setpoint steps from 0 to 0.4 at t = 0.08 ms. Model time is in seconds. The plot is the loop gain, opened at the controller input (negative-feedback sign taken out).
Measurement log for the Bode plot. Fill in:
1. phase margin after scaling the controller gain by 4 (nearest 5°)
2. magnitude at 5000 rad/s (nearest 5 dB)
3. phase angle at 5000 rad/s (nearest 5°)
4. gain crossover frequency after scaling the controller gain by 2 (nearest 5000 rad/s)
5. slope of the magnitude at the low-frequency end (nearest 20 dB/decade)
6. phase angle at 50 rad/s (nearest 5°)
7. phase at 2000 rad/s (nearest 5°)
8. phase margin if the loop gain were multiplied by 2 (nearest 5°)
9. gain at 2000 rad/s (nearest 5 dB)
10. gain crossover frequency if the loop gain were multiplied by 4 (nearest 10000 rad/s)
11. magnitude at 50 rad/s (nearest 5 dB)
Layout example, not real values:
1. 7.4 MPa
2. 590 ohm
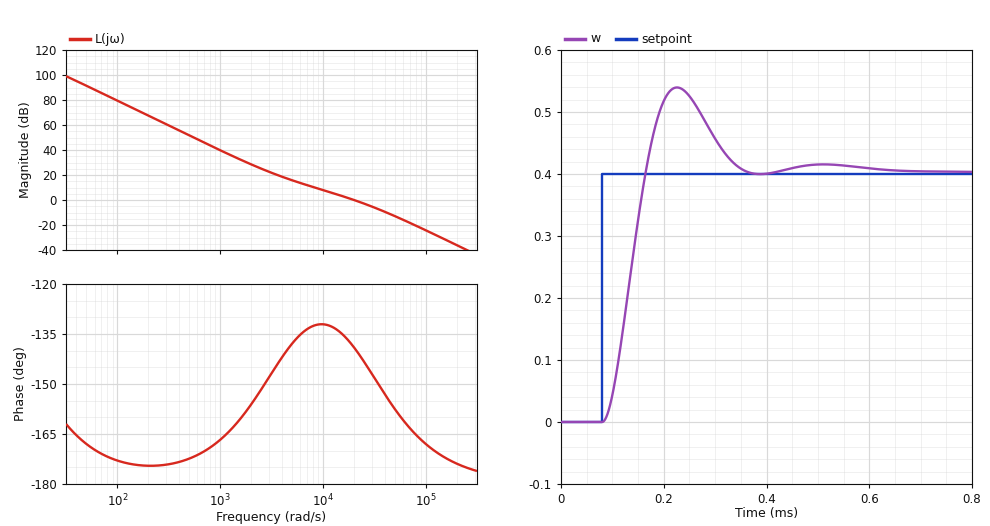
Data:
1. 25°
2. 15 dB
3. -140°
4. 30000 rad/s
5. -40 dB/decade
6. -170°
7. -155°
8. 30°
9. 30 dB
10. 50000 rad/s
11. 90 dB
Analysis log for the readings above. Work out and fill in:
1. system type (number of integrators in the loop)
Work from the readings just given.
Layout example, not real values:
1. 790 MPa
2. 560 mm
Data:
1. 2
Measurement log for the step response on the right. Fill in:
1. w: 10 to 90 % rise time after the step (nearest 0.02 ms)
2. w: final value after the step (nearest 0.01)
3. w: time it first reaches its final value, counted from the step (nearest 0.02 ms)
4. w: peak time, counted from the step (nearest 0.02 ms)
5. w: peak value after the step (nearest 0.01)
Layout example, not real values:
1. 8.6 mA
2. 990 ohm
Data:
1. 0.06 ms
2. 0.40
3. 0.08 ms
4. 0.14 ms
5. 0.54
